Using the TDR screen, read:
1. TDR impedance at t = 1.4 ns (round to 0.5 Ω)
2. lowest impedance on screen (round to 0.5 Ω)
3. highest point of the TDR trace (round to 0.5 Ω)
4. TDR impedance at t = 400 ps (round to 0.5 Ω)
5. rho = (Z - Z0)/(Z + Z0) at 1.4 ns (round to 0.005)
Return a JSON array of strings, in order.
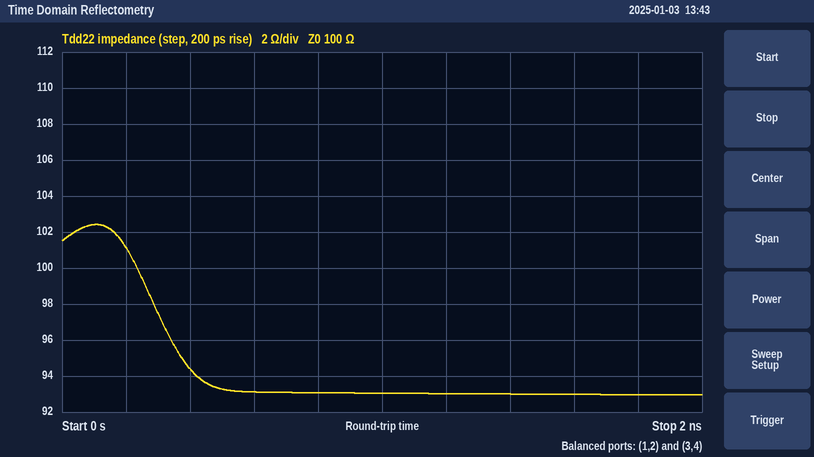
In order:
["93.0 Ω", "93.0 Ω", "102.5 Ω", "94.5 Ω", "-0.035"]
